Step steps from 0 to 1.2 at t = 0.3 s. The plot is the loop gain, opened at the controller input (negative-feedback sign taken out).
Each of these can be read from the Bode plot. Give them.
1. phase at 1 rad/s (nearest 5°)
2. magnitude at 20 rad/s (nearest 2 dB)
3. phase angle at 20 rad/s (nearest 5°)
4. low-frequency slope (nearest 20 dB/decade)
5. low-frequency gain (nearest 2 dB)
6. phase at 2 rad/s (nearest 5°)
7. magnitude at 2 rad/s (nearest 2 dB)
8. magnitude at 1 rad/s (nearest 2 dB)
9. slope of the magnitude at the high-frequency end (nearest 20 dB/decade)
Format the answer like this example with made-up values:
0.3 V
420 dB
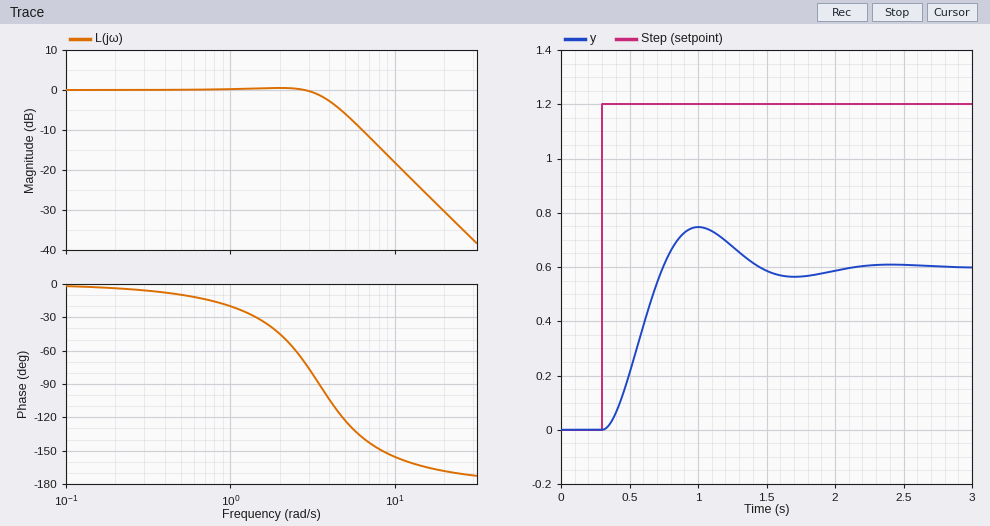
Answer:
-20°
-30 dB
-170°
0 dB/decade
0 dB
-45°
0 dB
0 dB
-40 dB/decade
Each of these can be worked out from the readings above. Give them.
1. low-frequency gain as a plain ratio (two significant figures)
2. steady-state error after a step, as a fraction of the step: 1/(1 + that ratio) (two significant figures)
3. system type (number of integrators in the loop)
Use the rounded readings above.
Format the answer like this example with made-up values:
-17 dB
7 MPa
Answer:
1.0
0.50
0
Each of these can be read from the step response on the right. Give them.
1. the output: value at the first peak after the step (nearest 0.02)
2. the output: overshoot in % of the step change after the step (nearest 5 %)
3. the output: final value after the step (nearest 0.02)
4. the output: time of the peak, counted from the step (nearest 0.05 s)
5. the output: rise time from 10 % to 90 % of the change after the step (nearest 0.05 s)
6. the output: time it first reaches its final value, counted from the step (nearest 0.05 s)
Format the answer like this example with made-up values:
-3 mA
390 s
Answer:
0.74
25 %
0.60
0.70 s
0.30 s
0.45 s
